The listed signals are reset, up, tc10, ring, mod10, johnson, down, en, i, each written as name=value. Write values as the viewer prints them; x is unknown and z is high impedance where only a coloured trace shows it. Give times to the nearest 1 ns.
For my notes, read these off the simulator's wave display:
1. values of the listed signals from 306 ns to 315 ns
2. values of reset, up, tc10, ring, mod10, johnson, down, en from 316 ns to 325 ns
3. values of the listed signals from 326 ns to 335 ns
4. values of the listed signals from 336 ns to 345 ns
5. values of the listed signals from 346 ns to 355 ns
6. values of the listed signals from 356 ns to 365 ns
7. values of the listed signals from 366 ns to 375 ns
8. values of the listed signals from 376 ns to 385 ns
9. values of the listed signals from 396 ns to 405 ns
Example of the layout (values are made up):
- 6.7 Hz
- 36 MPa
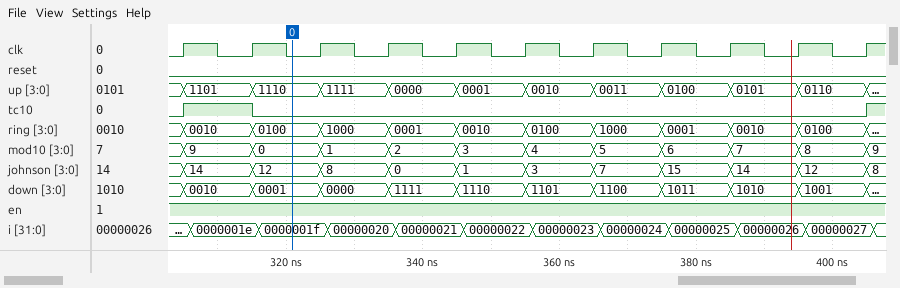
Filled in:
- reset=0, up=1101, tc10=1, ring=0010, mod10=9, johnson=14, down=0010, en=1, i=0000001e
- reset=0, up=1110, tc10=0, ring=0100, mod10=0, johnson=12, down=0001, en=1
- reset=0, up=1111, tc10=0, ring=1000, mod10=1, johnson=8, down=0000, en=1, i=00000020
- reset=0, up=0000, tc10=0, ring=0001, mod10=2, johnson=0, down=1111, en=1, i=00000021
- reset=0, up=0001, tc10=0, ring=0010, mod10=3, johnson=1, down=1110, en=1, i=00000022
- reset=0, up=0010, tc10=0, ring=0100, mod10=4, johnson=3, down=1101, en=1, i=00000023
- reset=0, up=0011, tc10=0, ring=1000, mod10=5, johnson=7, down=1100, en=1, i=00000024
- reset=0, up=0100, tc10=0, ring=0001, mod10=6, johnson=15, down=1011, en=1, i=00000025
- reset=0, up=0110, tc10=0, ring=0100, mod10=8, johnson=12, down=1001, en=1, i=00000027
